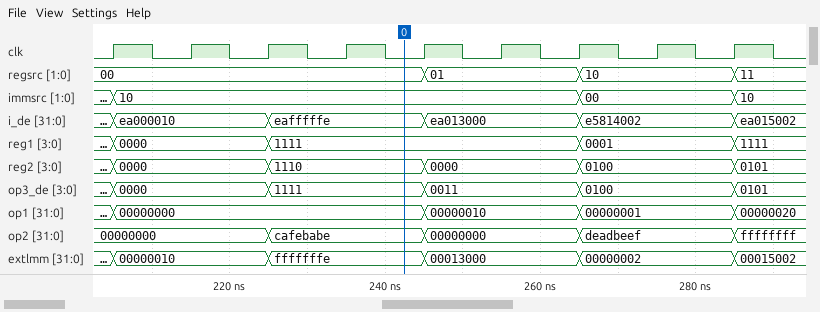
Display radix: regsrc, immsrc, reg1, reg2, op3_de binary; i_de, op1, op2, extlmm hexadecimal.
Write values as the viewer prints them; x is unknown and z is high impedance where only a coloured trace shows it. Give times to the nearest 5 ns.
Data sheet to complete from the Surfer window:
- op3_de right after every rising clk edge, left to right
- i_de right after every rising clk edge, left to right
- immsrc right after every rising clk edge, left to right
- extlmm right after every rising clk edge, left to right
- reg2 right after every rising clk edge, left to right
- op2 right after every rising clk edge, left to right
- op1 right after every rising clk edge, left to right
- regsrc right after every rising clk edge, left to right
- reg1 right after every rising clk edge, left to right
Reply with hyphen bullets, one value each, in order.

- 0000, 0000, 1111, 1111, 0011, 0011, 0100, 0100, 0101
- ea000010, ea000010, eafffffe, eafffffe, ea013000, ea013000, e5814002, e5814002, ea015002
- 10, 10, 10, 10, 10, 10, 00, 00, 10
- 00000010, 00000010, fffffffe, fffffffe, 00013000, 00013000, 00000002, 00000002, 00015002
- 0000, 0000, 1110, 1110, 0000, 0000, 0100, 0100, 0101
- 00000000, 00000000, cafebabe, cafebabe, 00000000, 00000000, deadbeef, deadbeef, ffffffff
- 00000000, 00000000, 00000000, 00000000, 00000010, 00000010, 00000001, 00000001, 00000020
- 00, 00, 00, 00, 01, 01, 10, 10, 11
- 0000, 0000, 1111, 1111, 1111, 1111, 0001, 0001, 1111
